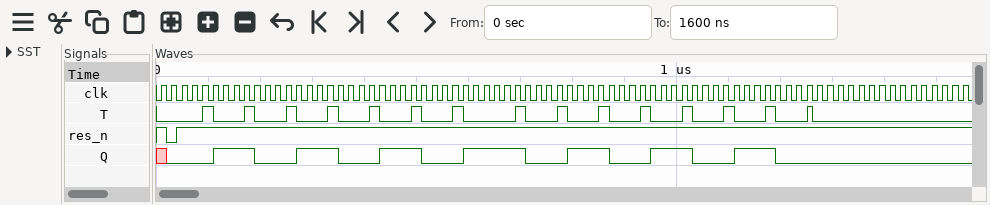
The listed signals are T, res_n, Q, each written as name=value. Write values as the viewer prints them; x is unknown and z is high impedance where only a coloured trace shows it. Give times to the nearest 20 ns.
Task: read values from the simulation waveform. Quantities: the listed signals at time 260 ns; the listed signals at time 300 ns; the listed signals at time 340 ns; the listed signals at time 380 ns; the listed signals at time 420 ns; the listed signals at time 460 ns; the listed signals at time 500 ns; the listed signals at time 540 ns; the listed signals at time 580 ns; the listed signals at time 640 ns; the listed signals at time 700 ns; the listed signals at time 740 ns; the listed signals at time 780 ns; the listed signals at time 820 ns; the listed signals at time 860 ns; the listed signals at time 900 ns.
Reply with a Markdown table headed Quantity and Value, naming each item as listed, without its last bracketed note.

| Quantity | Value |
|---|---|
| the listed signals at time 260 ns | T=1, res_n=1, Q=0 |
| the listed signals at time 300 ns | T=0, res_n=1, Q=1 |
| the listed signals at time 340 ns | T=1, res_n=1, Q=1 |
| the listed signals at time 380 ns | T=0, res_n=1, Q=0 |
| the listed signals at time 420 ns | T=1, res_n=1, Q=0 |
| the listed signals at time 460 ns | T=0, res_n=1, Q=1 |
| the listed signals at time 500 ns | T=1, res_n=1, Q=1 |
| the listed signals at time 540 ns | T=0, res_n=1, Q=0 |
| the listed signals at time 580 ns | T=1, res_n=1, Q=0 |
| the listed signals at time 640 ns | T=0, res_n=1, Q=1 |
| the listed signals at time 700 ns | T=1, res_n=1, Q=1 |
| the listed signals at time 740 ns | T=0, res_n=1, Q=0 |
| the listed signals at time 780 ns | T=1, res_n=1, Q=0 |
| the listed signals at time 820 ns | T=0, res_n=1, Q=1 |
| the listed signals at time 860 ns | T=1, res_n=1, Q=1 |
| the listed signals at time 900 ns | T=0, res_n=1, Q=0 |
